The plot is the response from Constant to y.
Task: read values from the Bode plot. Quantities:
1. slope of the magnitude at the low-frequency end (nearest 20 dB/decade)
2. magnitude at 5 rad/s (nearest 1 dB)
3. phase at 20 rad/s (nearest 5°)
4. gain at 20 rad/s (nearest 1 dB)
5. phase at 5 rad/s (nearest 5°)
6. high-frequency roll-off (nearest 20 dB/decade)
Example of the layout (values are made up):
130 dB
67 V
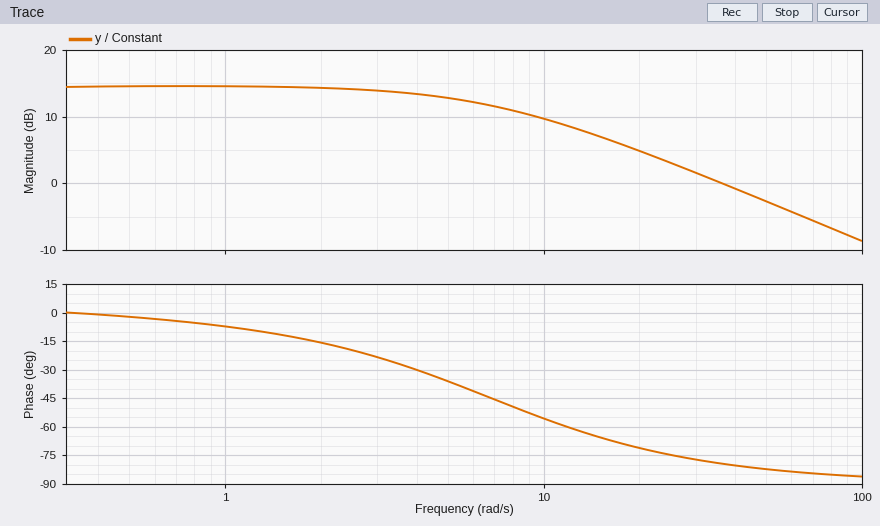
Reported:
0 dB/decade
13 dB
-70°
5 dB
-35°
-20 dB/decade
